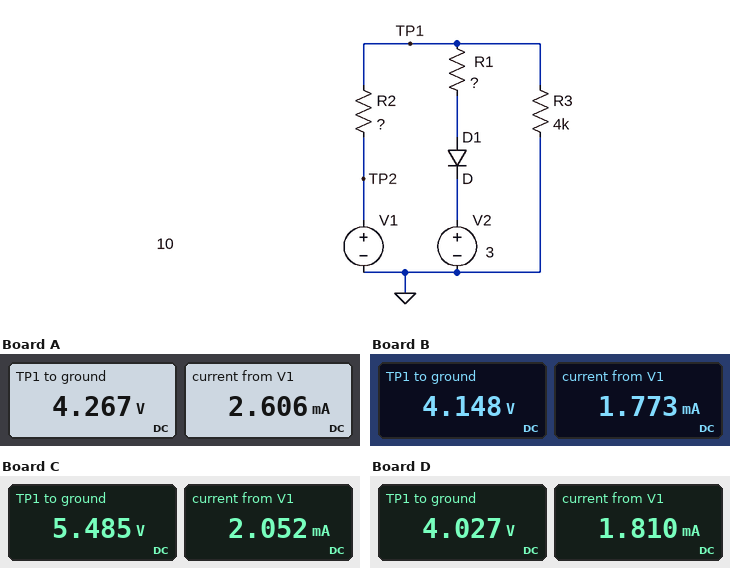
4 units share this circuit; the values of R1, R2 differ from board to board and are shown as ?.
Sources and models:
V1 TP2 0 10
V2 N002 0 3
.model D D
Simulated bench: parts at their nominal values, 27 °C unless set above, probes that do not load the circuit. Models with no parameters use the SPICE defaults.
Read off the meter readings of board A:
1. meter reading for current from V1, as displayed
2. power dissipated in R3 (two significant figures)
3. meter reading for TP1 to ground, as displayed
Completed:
2.606 mA
4.6 mW
4.267 V
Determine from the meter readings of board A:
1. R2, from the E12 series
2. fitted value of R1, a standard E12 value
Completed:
2.2 kΩ
390 Ω
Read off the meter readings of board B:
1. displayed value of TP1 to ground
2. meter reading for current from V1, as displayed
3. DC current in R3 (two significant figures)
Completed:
4.148 V
1.773 mA
1.0 mA
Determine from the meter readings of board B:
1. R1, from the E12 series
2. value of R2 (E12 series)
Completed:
680 Ω
3.3 kΩ
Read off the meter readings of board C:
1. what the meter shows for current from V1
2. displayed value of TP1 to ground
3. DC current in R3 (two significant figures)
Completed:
2.052 mA
5.485 V
1.4 mA
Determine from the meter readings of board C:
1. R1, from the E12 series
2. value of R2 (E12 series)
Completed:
2.7 kΩ
2.2 kΩ
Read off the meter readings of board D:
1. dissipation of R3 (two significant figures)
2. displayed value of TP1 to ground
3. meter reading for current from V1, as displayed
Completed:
4.1 mW
4.027 V
1.810 mA
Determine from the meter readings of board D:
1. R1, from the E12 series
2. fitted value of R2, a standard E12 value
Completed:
470 Ω
3.3 kΩ
